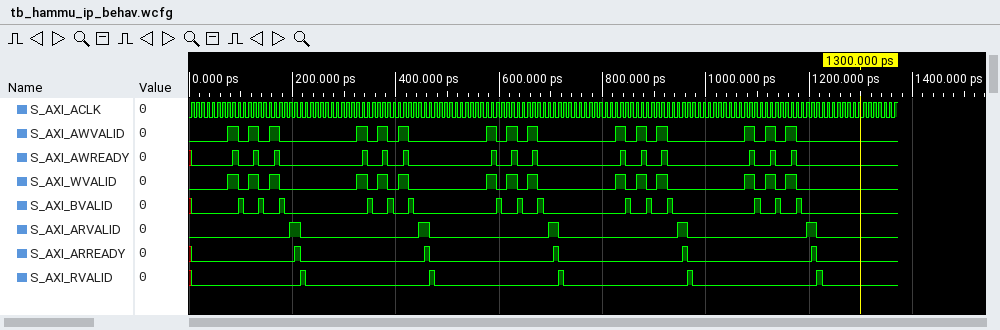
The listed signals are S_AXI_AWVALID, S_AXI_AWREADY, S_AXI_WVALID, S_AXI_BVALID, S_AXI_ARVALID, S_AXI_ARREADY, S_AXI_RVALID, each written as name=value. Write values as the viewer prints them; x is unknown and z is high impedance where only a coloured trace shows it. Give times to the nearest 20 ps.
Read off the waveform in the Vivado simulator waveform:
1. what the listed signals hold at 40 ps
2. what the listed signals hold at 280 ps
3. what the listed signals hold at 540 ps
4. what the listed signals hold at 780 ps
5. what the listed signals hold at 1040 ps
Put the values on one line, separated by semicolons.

S_AXI_AWVALID=0, S_AXI_AWREADY=0, S_AXI_WVALID=0, S_AXI_BVALID=0, S_AXI_ARVALID=0, S_AXI_ARREADY=0, S_AXI_RVALID=0; S_AXI_AWVALID=0, S_AXI_AWREADY=0, S_AXI_WVALID=0, S_AXI_BVALID=0, S_AXI_ARVALID=0, S_AXI_ARREADY=0, S_AXI_RVALID=0; S_AXI_AWVALID=0, S_AXI_AWREADY=0, S_AXI_WVALID=0, S_AXI_BVALID=0, S_AXI_ARVALID=0, S_AXI_ARREADY=0, S_AXI_RVALID=0; S_AXI_AWVALID=0, S_AXI_AWREADY=0, S_AXI_WVALID=0, S_AXI_BVALID=0, S_AXI_ARVALID=0, S_AXI_ARREADY=0, S_AXI_RVALID=0; S_AXI_AWVALID=0, S_AXI_AWREADY=0, S_AXI_WVALID=0, S_AXI_BVALID=0, S_AXI_ARVALID=0, S_AXI_ARREADY=0, S_AXI_RVALID=0
